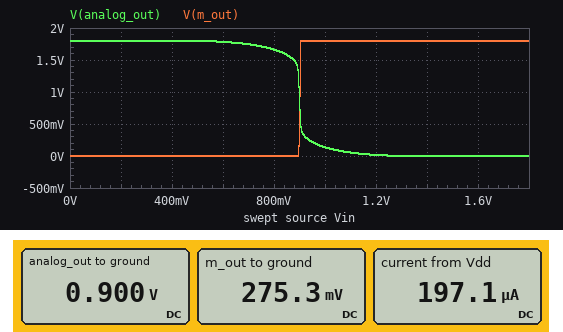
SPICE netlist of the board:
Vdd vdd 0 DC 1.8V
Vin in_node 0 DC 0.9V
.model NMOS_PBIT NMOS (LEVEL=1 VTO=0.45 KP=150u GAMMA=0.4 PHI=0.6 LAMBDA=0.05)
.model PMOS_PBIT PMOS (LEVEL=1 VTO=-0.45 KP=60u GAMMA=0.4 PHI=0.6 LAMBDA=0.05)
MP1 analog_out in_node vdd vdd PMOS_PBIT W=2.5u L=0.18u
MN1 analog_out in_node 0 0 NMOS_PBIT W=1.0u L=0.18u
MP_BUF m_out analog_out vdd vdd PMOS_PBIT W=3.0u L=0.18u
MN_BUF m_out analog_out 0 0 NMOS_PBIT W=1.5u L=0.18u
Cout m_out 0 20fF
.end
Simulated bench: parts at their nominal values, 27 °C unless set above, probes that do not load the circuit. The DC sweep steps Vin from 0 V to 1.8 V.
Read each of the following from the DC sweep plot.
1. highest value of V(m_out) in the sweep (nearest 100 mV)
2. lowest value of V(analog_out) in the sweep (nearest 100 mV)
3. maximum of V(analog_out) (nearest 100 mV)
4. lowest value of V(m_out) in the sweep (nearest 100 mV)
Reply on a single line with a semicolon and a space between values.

1.8 V; 0 V; 1.8 V; 0 V
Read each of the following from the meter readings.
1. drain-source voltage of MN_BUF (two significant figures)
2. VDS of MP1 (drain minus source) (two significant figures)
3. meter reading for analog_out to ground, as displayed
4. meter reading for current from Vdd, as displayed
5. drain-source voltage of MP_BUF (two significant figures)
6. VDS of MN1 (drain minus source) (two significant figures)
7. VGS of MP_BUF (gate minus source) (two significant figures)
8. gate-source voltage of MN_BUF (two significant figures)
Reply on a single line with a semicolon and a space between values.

280 mV; -900 mV; 0.900 V; 197.1 µA; -1.5 V; 900 mV; -900 mV; 900 mV
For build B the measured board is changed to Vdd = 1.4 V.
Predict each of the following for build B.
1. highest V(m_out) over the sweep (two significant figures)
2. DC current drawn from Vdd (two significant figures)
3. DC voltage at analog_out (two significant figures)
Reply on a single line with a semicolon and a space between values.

1.4 V; 1.1 µA; 3.0 mV
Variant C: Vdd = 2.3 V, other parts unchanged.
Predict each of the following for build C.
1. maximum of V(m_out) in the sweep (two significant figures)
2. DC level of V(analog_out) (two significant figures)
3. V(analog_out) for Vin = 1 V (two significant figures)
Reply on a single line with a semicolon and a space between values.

2.3 V; 2.2 V; 2.1 V
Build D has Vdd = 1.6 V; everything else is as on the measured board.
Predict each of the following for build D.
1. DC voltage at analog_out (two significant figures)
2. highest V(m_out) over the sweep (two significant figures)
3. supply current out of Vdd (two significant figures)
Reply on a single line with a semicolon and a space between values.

82 mV; 1.6 V; 28 µA
